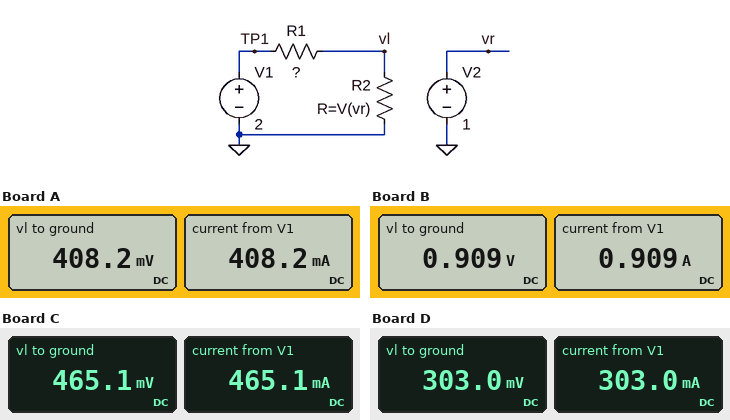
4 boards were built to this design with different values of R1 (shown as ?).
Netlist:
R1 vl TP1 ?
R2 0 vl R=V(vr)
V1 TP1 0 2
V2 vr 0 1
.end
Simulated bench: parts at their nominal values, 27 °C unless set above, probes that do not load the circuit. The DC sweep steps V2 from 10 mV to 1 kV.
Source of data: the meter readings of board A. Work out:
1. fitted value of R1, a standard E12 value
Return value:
3.9 Ω
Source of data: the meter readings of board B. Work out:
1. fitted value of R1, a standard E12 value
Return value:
1.2 Ω
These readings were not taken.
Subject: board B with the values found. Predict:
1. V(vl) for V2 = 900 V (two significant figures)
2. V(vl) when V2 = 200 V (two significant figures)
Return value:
2.0 V
2.0 V
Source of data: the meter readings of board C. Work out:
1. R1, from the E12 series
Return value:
3.3 Ω
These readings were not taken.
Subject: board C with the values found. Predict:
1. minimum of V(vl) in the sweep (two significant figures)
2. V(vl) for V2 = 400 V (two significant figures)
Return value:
6.0 mV
2.0 V
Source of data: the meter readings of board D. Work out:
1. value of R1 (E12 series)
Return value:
5.6 Ω
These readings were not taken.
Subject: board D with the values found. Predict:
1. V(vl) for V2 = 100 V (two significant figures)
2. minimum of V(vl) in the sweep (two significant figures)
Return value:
1.9 V
3.6 mV
